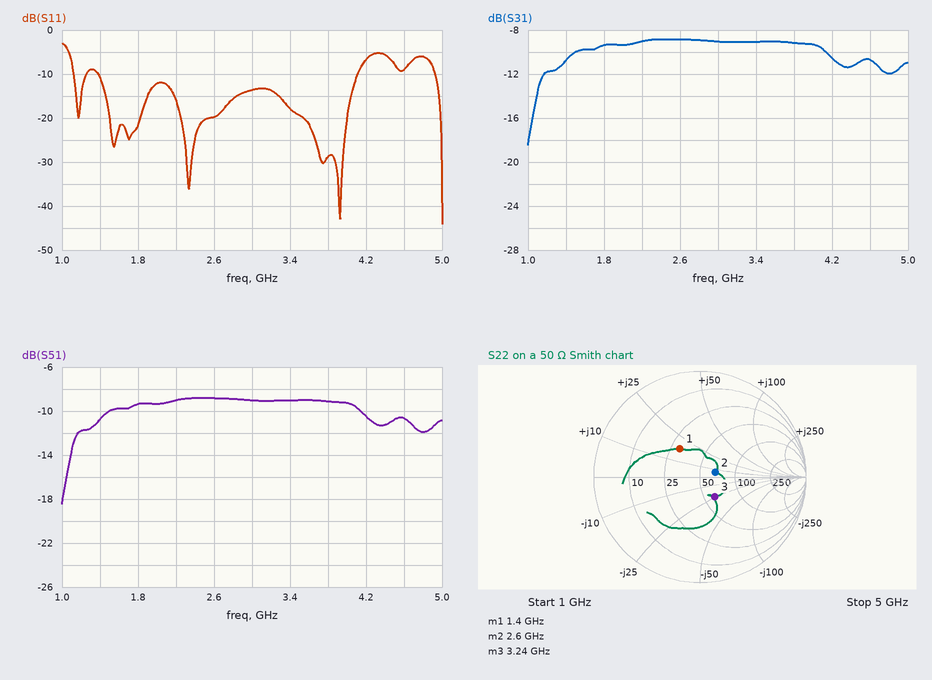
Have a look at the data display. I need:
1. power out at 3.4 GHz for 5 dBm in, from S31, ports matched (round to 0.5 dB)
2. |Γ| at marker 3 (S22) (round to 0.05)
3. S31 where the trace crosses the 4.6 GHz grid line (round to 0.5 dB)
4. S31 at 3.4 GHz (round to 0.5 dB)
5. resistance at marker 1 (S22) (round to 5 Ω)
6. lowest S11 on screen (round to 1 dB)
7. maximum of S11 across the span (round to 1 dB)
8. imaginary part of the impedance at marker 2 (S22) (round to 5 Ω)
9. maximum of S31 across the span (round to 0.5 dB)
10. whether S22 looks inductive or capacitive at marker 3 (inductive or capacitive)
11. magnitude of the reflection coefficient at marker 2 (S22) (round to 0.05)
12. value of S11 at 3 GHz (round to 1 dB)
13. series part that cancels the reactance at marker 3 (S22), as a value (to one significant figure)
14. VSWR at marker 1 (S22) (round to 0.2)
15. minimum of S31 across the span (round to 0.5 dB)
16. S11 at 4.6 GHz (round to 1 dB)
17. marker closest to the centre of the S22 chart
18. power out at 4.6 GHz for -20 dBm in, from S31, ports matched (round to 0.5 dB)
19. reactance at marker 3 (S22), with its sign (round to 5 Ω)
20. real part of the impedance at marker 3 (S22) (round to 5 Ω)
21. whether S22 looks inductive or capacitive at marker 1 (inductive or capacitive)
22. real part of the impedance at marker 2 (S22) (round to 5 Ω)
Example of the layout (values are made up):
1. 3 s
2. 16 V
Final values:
1. -4.0 dBm
2. 0.25
3. -10.5 dB
4. -9.0 dB
5. 30 Ω
6. -44 dB
7. -3 dB
8. +5 Ω
9. -9.0 dB
10. capacitive
11. 0.15
12. -14 dB
13. 1 nH
14. 2.0
15. -18.5 dB
16. -9 dB
17. marker 2
18. -30.5 dBm
19. -25 Ω
20. 60 Ω
21. inductive
22. 65 Ω
